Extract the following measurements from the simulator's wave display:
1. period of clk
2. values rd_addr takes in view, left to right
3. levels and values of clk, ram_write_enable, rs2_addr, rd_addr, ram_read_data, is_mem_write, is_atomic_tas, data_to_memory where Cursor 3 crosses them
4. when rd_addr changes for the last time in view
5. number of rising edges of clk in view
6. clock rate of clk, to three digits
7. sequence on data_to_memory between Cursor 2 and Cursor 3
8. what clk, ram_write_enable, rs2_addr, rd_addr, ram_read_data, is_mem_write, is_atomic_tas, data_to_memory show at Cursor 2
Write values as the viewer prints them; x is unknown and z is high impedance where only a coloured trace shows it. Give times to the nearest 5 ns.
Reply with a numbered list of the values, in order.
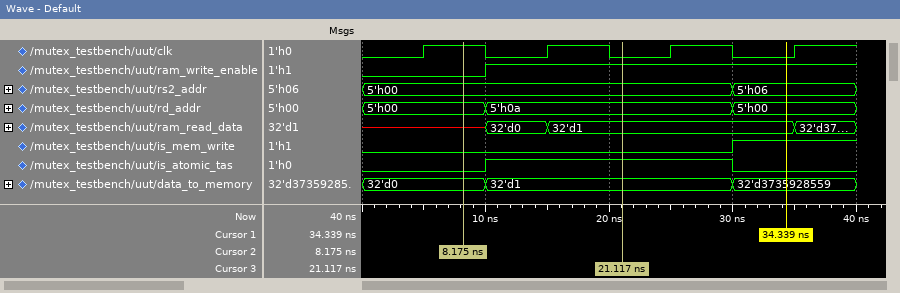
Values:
1. 10 ns
2. 5'h00, 5'h0a, 5'h00
3. clk=0, ram_write_enable=1, rs2_addr=5'h00, rd_addr=5'h0a, ram_read_data=32'd1, is_mem_write=0, is_atomic_tas=1, data_to_memory=32'd1
4. 30 ns
5. 4
6. 100 MHz
7. 32'd0, 32'd1
8. clk=1, ram_write_enable=0, rs2_addr=5'h00, rd_addr=5'h00, ram_read_data=x, is_mem_write=0, is_atomic_tas=0, data_to_memory=32'd0
